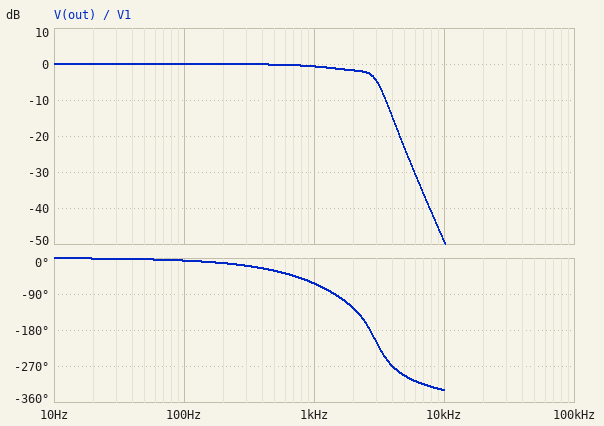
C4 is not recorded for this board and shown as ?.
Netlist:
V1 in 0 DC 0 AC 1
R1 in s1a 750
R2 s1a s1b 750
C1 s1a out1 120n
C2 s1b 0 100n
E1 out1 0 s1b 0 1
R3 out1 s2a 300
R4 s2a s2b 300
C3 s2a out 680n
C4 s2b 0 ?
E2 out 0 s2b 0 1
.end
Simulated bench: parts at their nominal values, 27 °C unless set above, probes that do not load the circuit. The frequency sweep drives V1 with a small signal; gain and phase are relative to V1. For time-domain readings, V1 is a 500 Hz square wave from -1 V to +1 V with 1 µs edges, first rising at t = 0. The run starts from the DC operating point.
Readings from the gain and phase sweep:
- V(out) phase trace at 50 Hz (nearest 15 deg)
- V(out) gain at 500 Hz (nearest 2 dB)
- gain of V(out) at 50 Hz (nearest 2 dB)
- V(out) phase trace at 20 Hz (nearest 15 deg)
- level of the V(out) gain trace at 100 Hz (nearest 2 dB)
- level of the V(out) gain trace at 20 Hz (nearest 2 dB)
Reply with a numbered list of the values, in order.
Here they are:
1. 0 deg
2. 0 dB
3. 0 dB
4. 0 deg
5. 0 dB
6. 0 dB
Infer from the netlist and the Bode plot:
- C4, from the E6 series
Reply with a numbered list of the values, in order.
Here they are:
1. 47 nF
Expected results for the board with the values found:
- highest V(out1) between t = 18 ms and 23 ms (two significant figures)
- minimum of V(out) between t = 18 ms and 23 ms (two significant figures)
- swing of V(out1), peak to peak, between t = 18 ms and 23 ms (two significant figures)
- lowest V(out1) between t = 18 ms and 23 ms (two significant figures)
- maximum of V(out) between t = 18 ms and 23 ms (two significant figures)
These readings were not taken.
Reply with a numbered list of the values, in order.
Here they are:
1. 1.0 V
2. -1.1 V
3. 2.0 V
4. -1.0 V
5. 1.1 V
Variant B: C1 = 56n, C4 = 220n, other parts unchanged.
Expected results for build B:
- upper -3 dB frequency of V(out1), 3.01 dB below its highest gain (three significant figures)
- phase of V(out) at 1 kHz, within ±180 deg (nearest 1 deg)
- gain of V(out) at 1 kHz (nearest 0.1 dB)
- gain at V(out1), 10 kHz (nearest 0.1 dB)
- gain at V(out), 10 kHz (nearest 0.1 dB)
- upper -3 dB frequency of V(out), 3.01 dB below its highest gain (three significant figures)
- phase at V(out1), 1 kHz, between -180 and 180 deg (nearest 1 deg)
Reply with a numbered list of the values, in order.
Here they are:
1. 1.23 kHz
2. -108 deg
3. -1.8 dB
4. -23.4 dB
5. -57.9 dB
6. 1.19 kHz
7. -47 deg
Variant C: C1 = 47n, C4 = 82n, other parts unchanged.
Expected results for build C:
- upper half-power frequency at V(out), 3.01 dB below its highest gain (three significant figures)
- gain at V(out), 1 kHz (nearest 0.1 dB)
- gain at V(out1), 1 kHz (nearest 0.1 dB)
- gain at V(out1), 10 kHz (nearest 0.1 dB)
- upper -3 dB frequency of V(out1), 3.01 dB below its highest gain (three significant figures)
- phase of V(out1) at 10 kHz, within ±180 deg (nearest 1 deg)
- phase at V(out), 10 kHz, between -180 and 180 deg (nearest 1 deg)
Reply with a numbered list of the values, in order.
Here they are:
1. 2.16 kHz
2. -1.0 dB
3. -2.3 dB
4. -22.5 dB
5. 1.20 kHz
6. -135 deg
7. 54 deg
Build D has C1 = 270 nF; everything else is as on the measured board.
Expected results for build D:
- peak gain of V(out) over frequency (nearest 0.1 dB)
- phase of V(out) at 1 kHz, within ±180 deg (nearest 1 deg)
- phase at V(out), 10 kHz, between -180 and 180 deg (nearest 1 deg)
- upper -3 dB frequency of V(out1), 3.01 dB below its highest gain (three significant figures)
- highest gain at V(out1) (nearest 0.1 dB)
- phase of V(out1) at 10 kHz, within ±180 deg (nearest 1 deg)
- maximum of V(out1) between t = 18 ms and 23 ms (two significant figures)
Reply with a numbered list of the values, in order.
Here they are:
1. 0.8 dB
2. -78 deg
3. 19 deg
4. 1.43 kHz
5. 0.3 dB
6. -171 deg
7. 1.2 V
